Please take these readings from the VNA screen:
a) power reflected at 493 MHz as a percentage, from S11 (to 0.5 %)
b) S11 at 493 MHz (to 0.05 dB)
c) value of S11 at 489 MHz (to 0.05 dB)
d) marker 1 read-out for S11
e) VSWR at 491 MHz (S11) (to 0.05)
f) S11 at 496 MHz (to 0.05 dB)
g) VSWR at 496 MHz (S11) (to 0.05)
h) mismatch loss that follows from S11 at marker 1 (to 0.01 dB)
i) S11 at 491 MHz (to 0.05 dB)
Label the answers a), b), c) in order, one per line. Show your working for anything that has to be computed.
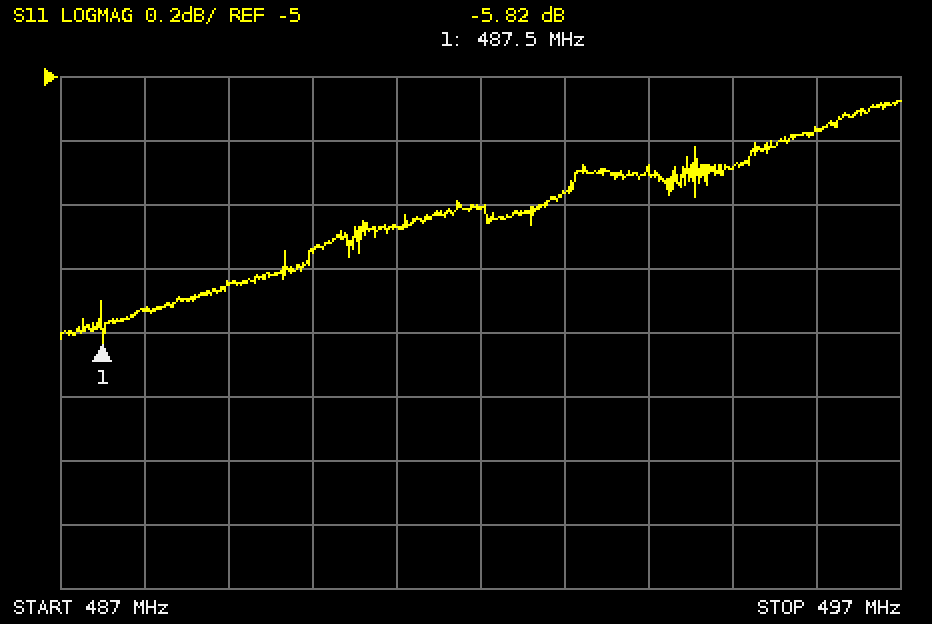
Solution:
a) 10^(-5.35/10) ≈ 29.2 %, so 29.0 % to the nearest 0.5 %
b) -5.35 dB
c) -5.65 dB
d) -5.82 dB
e) |Γ| = 10^(-5.45/20) = 0.5339; VSWR = (1 + 0.5339)/(1 − 0.5339) ≈ 3.29, so 3.30 to the nearest 0.05
f) -5.15 dB
g) |Γ| = 10^(-5.15/20) = 0.5527; VSWR = (1 + 0.5527)/(1 − 0.5527) ≈ 3.47, so 3.45 to the nearest 0.05
h) −10 log10(1 − 10^(-5.82/10)) ≈ 1.32 dB
i) -5.45 dB
